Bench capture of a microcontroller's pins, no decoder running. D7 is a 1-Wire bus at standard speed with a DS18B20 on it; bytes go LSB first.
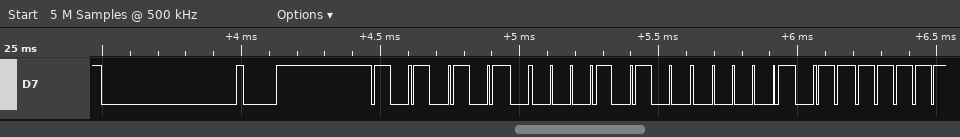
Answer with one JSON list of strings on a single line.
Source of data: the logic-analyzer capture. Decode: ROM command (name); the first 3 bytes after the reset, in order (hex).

["Match ROM", "55 28 D0"]
